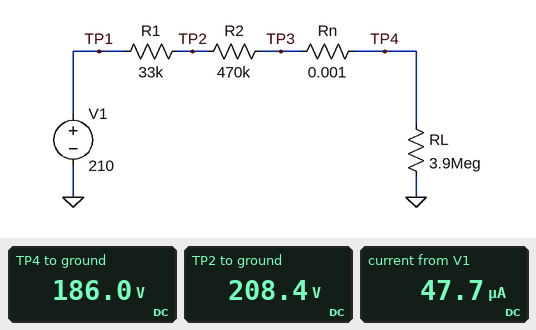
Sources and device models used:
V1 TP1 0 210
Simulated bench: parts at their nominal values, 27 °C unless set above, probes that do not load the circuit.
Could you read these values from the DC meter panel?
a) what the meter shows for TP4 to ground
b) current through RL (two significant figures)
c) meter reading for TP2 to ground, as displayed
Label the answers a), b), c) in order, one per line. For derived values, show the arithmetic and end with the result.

a) 186.0 V
b) (186 V) / 3.9 MΩ = 48 µA
c) 208.4 V
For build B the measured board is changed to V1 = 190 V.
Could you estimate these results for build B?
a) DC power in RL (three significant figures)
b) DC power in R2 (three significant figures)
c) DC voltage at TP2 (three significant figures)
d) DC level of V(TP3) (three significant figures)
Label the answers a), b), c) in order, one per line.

a) 7.26 mW
b) 875 µW
c) 189 V
d) 168 V
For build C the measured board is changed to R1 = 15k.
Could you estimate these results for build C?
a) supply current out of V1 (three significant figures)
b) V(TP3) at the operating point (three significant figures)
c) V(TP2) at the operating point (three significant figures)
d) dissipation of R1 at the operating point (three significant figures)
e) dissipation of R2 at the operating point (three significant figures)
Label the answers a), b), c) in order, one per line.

a) 47.9 µA
b) 187 V
c) 209 V
d) 34.4 µW
e) 1.08 mW
